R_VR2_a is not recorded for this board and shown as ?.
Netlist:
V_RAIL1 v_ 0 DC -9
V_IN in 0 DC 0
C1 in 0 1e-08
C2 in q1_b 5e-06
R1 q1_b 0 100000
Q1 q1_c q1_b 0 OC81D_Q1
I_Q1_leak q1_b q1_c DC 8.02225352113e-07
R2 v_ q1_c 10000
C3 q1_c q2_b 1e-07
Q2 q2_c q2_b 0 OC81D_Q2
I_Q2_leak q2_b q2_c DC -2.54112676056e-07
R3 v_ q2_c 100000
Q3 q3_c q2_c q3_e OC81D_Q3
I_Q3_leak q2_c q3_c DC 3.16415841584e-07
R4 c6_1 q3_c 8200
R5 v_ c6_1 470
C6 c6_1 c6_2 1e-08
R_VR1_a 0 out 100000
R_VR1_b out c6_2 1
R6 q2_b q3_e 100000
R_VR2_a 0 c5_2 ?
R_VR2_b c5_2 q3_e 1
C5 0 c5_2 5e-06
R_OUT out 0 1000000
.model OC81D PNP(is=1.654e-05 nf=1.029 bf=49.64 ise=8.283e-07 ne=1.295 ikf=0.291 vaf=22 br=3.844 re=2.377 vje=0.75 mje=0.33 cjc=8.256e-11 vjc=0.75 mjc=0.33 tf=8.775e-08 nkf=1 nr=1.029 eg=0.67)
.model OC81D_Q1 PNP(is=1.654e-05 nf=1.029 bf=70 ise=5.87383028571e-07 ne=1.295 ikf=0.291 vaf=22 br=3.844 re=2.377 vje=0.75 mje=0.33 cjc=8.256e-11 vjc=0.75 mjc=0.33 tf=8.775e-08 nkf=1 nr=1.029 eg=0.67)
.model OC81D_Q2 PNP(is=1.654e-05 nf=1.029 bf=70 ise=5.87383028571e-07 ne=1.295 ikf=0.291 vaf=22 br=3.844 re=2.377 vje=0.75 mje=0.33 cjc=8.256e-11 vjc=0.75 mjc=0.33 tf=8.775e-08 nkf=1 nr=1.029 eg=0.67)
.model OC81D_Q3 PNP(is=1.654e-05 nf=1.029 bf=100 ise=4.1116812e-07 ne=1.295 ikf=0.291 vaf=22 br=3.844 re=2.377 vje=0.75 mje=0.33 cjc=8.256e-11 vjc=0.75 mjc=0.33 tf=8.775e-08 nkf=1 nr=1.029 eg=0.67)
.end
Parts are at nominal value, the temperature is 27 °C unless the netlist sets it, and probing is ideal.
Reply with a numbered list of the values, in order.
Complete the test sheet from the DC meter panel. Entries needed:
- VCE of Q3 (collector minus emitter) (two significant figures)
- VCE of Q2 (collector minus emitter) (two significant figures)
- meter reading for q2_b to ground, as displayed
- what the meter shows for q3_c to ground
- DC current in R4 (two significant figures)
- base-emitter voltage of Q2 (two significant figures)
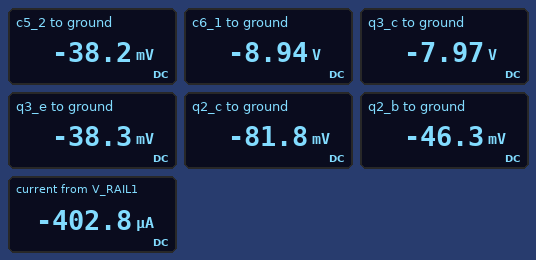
1. -7.9 V
2. -82 mV
3. -46.3 mV
4. -7.97 V
5. 120 µA
6. -46 mV
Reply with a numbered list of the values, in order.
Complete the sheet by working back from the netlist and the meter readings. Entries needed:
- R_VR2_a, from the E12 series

1. 330 Ω
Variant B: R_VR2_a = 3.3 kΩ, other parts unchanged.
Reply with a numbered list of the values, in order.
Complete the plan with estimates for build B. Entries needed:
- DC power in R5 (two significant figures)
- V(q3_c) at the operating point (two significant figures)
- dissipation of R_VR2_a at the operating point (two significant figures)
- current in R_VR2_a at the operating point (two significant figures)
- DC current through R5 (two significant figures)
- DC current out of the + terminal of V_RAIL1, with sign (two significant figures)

1. 370 nW
2. -8.8 V
3. 1.8 µW
4. 23 µA
5. 28 µA
6. -310 µA
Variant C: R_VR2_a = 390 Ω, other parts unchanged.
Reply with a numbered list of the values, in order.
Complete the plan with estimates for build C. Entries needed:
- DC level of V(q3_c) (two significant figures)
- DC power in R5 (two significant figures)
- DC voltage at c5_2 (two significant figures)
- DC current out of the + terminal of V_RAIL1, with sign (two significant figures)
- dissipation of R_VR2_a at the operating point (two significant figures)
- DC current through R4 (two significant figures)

1. -8.1 V
2. 5.4 µW
3. -41 mV
4. -390 µA
5. 4.3 µW
6. 110 µA
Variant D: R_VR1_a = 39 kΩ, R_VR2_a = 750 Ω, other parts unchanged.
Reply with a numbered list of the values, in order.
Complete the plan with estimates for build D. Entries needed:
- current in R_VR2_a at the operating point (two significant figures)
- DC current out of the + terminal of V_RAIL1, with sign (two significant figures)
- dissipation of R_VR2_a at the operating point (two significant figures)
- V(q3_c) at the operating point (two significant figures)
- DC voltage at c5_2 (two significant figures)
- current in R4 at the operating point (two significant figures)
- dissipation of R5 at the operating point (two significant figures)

1. 68 µA
2. -360 µA
3. 3.5 µW
4. -8.4 V
5. -51 mV
6. 72 µA
7. 2.4 µW
